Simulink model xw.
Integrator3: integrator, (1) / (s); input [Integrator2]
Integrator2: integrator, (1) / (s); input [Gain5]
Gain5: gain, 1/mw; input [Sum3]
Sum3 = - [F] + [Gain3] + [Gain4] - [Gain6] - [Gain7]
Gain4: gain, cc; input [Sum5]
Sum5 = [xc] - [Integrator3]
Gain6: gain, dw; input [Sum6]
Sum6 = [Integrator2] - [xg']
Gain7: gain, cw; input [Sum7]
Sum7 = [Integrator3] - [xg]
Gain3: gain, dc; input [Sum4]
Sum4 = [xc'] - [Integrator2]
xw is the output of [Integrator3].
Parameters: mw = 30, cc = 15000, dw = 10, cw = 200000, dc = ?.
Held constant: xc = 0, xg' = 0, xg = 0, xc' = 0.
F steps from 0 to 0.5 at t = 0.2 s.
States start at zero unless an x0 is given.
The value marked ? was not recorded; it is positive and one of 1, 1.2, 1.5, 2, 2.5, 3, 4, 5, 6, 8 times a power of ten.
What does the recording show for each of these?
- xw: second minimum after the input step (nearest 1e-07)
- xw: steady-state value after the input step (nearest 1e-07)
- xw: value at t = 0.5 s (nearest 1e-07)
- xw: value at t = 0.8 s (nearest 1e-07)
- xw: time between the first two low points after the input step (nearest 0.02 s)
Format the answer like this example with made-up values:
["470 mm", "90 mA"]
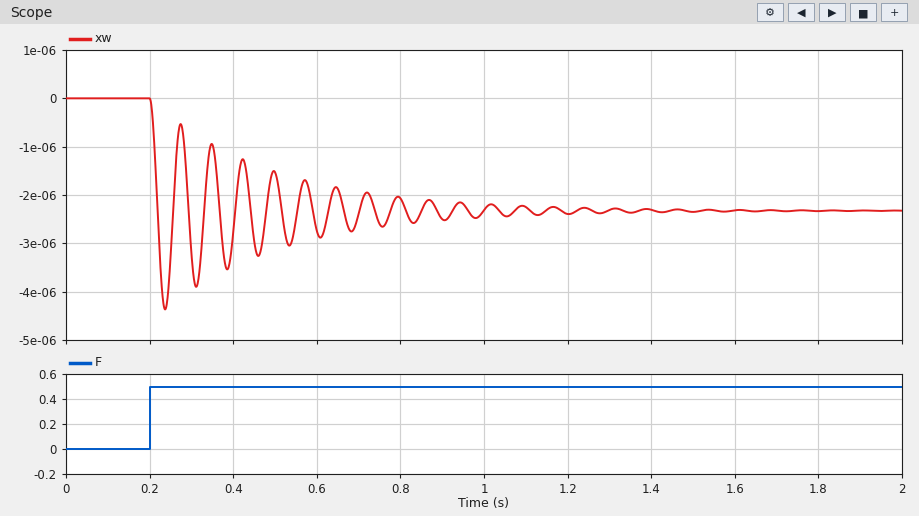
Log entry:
["-0.0000039", "-0.0000023", "-0.0000015", "-0.0000021", "0.08 s"]
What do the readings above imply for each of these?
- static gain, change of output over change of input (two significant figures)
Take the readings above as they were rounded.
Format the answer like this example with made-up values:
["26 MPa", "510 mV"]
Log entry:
["-0.0000046"]
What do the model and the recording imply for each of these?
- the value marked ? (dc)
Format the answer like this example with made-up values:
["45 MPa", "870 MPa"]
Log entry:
["200"]
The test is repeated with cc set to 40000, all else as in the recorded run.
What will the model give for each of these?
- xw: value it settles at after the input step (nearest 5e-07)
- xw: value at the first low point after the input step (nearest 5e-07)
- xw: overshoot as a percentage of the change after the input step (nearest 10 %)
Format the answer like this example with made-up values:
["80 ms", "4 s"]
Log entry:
["-0.0000020", "-0.0000040", "90 %"]
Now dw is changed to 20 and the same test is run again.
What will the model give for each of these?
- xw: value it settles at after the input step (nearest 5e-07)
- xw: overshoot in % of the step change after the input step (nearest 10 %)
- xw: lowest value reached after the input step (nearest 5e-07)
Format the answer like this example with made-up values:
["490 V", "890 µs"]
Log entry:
["-0.0000025", "90 %", "-0.0000045"]
